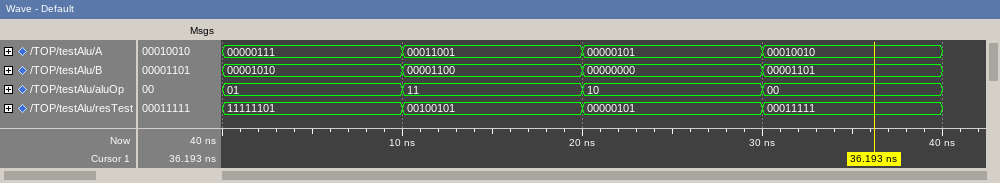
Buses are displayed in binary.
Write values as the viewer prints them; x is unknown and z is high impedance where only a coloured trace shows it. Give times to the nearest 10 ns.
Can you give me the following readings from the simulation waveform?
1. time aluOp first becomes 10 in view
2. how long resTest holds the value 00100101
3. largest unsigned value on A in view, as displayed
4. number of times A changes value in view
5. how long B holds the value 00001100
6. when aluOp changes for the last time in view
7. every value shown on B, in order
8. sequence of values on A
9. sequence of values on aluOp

20 ns
10 ns
00011001
3
10 ns
30 ns
00001010, 00001100, 00000000, 00001101
00000111, 00011001, 00000101, 00010010
01, 11, 10, 00
